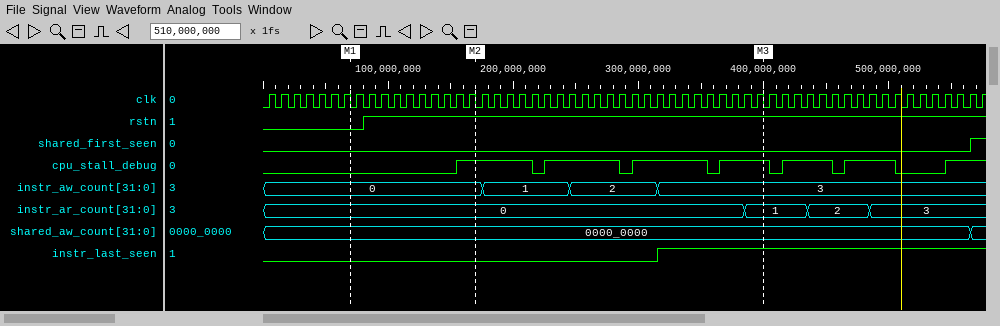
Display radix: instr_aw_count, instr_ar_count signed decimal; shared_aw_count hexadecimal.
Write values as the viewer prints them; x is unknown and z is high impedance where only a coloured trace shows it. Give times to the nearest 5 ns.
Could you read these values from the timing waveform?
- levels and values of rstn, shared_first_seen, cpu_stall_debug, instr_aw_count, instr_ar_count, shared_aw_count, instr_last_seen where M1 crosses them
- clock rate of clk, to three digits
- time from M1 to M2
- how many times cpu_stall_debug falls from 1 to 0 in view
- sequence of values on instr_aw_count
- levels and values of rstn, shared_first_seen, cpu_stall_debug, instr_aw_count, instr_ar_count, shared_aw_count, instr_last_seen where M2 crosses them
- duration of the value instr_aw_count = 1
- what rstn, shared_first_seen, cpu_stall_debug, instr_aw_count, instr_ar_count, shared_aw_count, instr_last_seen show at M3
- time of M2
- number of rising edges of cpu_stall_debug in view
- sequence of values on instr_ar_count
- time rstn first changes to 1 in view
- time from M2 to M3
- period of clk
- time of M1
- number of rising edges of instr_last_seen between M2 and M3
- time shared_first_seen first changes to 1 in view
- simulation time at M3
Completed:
rstn=0, shared_first_seen=0, cpu_stall_debug=0, instr_aw_count=0, instr_ar_count=0, shared_aw_count=0000_0000, instr_last_seen=0
100 MHz
100 ns
6
0, 1, 2, 3
rstn=1, shared_first_seen=0, cpu_stall_debug=1, instr_aw_count=0, instr_ar_count=0, shared_aw_count=0000_0000, instr_last_seen=0
70 ns
rstn=1, shared_first_seen=0, cpu_stall_debug=1, instr_aw_count=3, instr_ar_count=1, shared_aw_count=0000_0000, instr_last_seen=1
170 ns
7
0, 1, 2, 3
80 ns
230 ns
10 ns
70 ns
1
565 ns
400 ns
